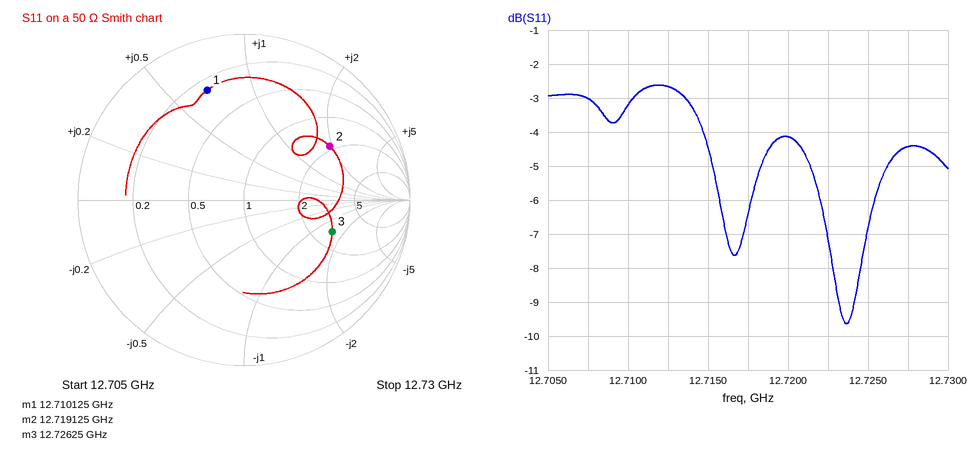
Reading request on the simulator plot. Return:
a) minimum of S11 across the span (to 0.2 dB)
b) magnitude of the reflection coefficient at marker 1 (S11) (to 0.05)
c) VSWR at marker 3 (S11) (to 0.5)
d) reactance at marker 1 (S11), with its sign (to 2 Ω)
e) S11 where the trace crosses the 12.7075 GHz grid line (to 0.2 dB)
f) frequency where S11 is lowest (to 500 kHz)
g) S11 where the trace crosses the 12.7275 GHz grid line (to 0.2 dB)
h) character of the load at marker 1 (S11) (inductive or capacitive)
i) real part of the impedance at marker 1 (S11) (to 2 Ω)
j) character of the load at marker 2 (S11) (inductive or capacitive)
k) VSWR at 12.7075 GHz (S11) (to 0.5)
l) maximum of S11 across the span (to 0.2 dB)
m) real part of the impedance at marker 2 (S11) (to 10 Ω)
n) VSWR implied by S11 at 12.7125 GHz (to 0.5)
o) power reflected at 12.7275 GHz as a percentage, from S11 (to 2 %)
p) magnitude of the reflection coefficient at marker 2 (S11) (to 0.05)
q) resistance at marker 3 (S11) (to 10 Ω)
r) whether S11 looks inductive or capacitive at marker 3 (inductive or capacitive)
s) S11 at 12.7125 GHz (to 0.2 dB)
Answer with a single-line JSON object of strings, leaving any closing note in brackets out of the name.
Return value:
{"minimum of S11 across the span": "-9.6 dB", "magnitude of the reflection coefficient at marker 1 (S11)": "0.70", "VSWR at marker 3 (S11)": "3.5", "reactance at marker 1 (S11), with its sign": "+34 Ω", "S11 where the trace crosses the 12.7075 GHz grid line": "-3.0 dB", "frequency where S11 is lowest": "12.7235 GHz", "S11 where the trace crosses the 12.7275 GHz grid line": "-4.4 dB", "character of the load at marker 1 (S11)": "inductive", "real part of the impedance at marker 1 (S11)": "14 Ω", "character of the load at marker 2 (S11)": "inductive", "VSWR at 12.7075 GHz (S11)": "6.0", "maximum of S11 across the span": "-2.6 dB", "real part of the impedance at marker 2 (S11)": "90 Ω", "VSWR implied by S11 at 12.7125 GHz": "6.5", "power reflected at 12.7275 GHz as a percentage, from S11": "36 %", "magnitude of the reflection coefficient at marker 2 (S11)": "0.60", "resistance at marker 3 (S11)": "130 Ω", "whether S11 looks inductive or capacitive at marker 3": "capacitive", "S11 at 12.7125 GHz": "-2.6 dB"}
